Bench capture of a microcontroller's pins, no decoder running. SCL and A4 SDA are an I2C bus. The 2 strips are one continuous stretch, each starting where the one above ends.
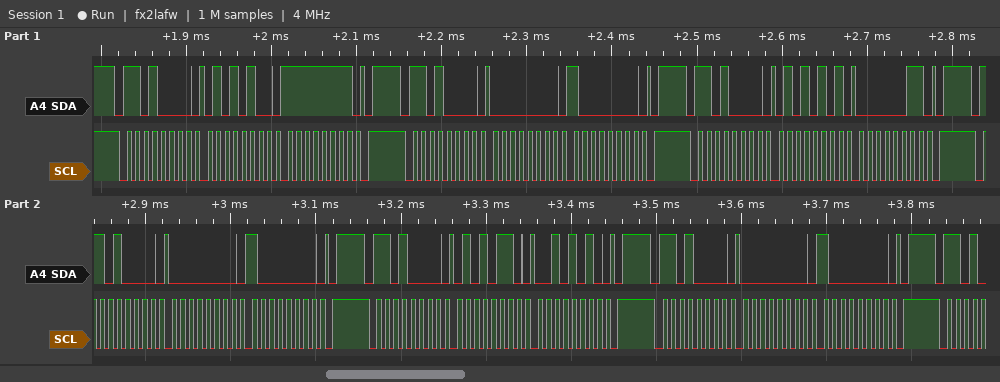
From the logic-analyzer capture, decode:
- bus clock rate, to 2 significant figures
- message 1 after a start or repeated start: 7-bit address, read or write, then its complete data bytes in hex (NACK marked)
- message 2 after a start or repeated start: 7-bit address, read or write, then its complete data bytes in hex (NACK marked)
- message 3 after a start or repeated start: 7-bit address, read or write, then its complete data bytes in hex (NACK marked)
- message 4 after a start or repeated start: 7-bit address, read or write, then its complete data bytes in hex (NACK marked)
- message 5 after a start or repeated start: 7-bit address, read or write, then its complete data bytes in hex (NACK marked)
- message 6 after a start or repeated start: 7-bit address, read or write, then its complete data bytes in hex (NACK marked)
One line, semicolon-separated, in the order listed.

100 kHz; 0x68 write: 54 FF; 0x68 write: 00 80; 0x68 write: 55 03; 0x68 write: 00 80; 0x68 write: 56 2A; 0x68 write: 00 80
